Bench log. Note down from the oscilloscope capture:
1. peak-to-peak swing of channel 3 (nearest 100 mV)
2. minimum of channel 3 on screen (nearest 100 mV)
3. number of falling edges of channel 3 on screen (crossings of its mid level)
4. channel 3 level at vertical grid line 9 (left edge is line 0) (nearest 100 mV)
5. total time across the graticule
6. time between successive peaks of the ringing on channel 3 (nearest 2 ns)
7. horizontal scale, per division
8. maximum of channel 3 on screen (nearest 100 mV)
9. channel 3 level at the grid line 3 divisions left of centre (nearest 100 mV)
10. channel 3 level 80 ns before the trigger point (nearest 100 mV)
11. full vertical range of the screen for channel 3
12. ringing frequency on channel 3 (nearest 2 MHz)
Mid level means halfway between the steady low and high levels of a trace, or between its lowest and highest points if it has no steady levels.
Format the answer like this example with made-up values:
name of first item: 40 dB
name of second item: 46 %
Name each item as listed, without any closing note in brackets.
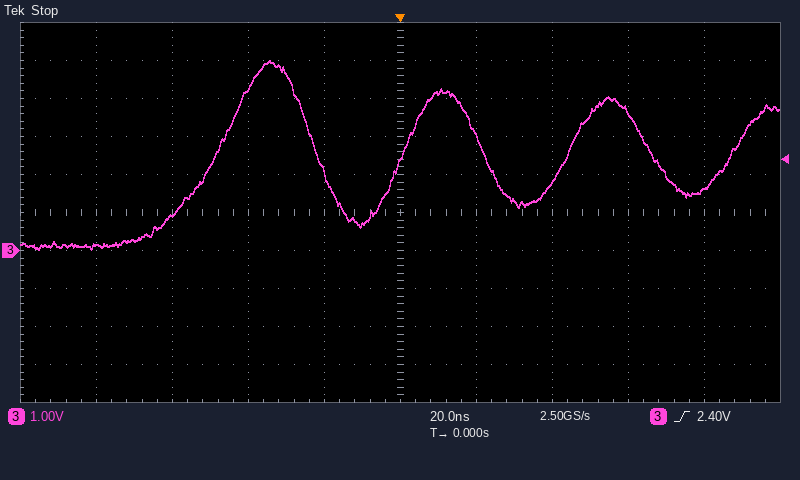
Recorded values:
peak-to-peak swing of channel 3: 5.0 V
minimum of channel 3 on screen: 0.0 V
number of falling edges of channel 3 on screen: 3
channel 3 level at vertical grid line 9 (left edge is line 0): 1.6 V
total time across the graticule: 200 ns
time between successive peaks of the ringing on channel 3: 44 ns
horizontal scale, per division: 20 ns
maximum of channel 3 on screen: 5.0 V
channel 3 level at the grid line 3 divisions left of centre: 900 mV
channel 3 level 80 ns before the trigger point: 100 mV
full vertical range of the screen for channel 3: 10 V
ringing frequency on channel 3: 22 MHz
